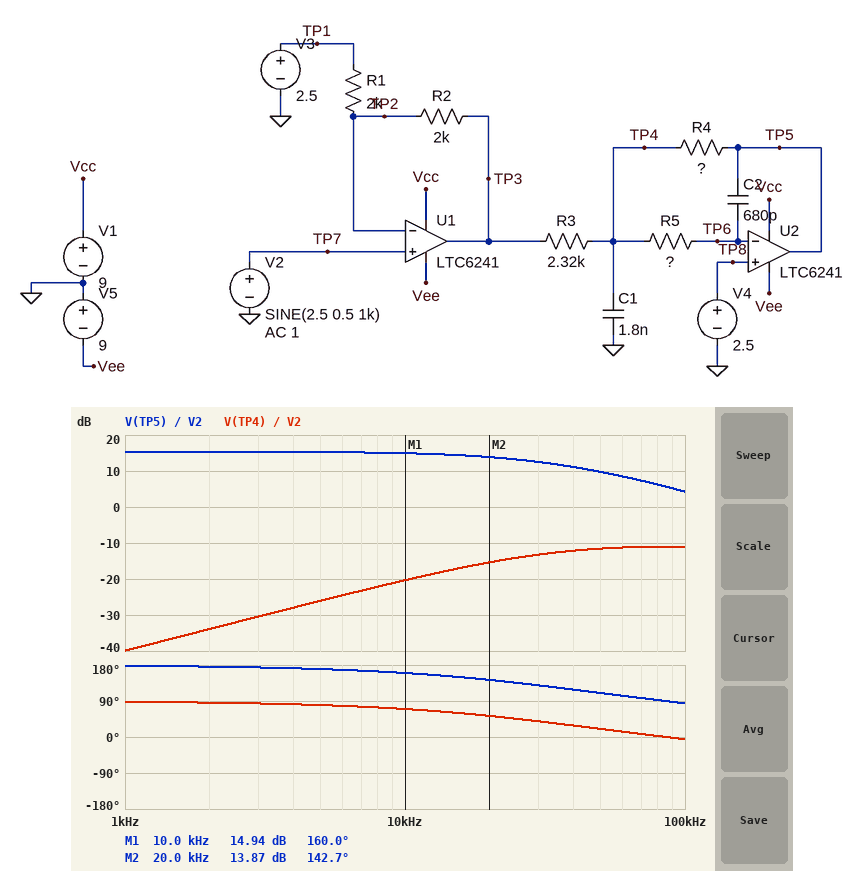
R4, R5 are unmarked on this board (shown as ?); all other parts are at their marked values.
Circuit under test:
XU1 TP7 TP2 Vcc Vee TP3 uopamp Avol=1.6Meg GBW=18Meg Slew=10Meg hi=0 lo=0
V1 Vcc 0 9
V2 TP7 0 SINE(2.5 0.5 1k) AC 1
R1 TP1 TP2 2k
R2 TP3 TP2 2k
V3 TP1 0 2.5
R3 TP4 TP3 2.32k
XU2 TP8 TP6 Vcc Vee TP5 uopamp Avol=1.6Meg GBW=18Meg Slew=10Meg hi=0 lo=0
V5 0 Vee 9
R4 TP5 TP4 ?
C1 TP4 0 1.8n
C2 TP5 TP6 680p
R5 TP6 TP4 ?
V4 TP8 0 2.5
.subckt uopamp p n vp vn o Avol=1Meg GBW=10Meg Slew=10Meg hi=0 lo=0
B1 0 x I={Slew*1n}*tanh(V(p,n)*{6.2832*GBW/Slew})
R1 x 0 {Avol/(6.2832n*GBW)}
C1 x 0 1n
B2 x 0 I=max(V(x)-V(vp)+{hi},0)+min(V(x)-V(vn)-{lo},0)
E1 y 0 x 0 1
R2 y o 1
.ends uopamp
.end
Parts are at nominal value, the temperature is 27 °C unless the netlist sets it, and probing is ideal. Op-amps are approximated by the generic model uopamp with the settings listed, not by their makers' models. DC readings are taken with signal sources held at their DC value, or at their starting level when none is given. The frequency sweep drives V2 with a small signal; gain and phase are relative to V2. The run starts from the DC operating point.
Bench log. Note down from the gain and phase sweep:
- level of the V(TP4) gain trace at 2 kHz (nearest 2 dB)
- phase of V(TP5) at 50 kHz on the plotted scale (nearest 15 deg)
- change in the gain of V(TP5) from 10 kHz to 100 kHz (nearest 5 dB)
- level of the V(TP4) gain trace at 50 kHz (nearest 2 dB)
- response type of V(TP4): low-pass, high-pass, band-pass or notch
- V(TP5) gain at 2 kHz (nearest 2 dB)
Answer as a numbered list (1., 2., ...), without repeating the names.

1. -34 dB
2. 105 deg
3. -10 dB
4. -12 dB
5. high-pass
6. 16 dB
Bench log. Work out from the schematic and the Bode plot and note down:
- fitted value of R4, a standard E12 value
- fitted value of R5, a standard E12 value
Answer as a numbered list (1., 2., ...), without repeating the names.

1. 6.8 kΩ
2. 390 Ω
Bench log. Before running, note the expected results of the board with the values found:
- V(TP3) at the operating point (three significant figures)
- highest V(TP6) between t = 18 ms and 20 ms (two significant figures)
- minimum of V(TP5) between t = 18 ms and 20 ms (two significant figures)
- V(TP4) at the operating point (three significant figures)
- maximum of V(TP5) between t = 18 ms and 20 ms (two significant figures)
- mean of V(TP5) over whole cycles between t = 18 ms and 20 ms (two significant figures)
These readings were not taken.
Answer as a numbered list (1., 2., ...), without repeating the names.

1. 2.50 V
2. 2.5 V
3. -430 mV
4. 2.50 V
5. 5.4 V
6. 2.5 V
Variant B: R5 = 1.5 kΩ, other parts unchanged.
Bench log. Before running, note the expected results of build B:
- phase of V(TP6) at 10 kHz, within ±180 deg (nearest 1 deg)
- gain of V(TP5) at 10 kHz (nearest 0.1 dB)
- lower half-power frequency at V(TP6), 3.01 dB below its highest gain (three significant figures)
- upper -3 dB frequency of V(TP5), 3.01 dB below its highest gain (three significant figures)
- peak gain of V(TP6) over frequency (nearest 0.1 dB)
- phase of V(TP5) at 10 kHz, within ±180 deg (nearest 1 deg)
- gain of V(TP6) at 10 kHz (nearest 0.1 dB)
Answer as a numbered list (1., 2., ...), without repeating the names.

1. 60 deg
2. 14.6 dB
3. 16.0 kHz
4. 21.9 kHz
5. -44.5 dB
6. 150 deg
7. -50.5 dB
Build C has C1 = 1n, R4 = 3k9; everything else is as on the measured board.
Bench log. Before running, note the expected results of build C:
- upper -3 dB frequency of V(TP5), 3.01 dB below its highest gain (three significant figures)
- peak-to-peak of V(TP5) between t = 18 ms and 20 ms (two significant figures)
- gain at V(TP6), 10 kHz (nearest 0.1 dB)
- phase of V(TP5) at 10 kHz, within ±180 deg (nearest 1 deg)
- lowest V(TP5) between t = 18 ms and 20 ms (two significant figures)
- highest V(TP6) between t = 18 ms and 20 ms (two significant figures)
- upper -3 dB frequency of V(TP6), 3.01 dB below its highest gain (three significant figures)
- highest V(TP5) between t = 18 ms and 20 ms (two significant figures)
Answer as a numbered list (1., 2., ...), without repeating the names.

1. 51.9 kHz
2. 3.4 V
3. -54.7 dB
4. 168 deg
5. 820 mV
6. 2.5 V
7. 544 kHz
8. 4.2 V
